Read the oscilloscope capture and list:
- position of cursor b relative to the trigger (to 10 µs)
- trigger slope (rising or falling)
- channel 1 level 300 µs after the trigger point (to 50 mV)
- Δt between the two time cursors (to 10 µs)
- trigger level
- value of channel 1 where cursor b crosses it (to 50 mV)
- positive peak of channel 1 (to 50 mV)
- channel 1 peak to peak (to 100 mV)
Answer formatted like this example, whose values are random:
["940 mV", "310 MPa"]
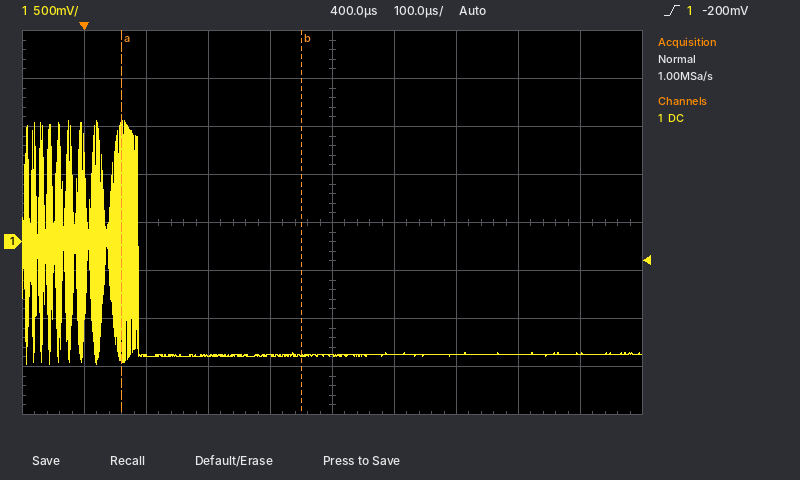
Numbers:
["+350 µs", "rising", "-1.20 V", "290 µs", "-200 mV", "-1.20 V", "1.25 V", "2.50 V"]
